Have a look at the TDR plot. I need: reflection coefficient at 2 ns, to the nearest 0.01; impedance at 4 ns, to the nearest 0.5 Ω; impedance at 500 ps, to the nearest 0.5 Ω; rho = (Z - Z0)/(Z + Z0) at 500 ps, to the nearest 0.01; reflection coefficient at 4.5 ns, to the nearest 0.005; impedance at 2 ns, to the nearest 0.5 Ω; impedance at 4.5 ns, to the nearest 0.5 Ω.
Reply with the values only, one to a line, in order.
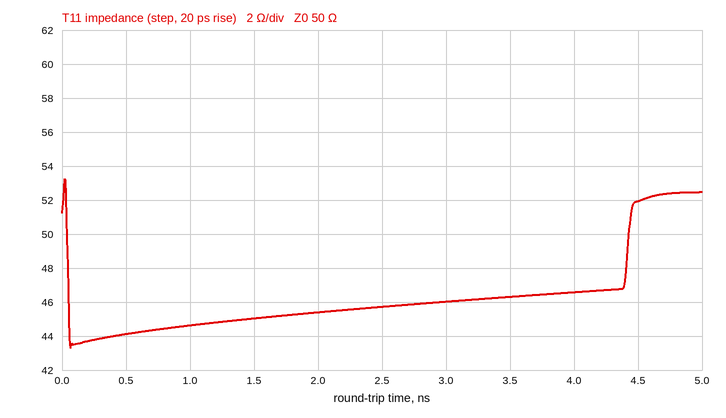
-0.05
46.5 Ω
44.0 Ω
-0.06
+0.020
45.5 Ω
52.0 Ω
